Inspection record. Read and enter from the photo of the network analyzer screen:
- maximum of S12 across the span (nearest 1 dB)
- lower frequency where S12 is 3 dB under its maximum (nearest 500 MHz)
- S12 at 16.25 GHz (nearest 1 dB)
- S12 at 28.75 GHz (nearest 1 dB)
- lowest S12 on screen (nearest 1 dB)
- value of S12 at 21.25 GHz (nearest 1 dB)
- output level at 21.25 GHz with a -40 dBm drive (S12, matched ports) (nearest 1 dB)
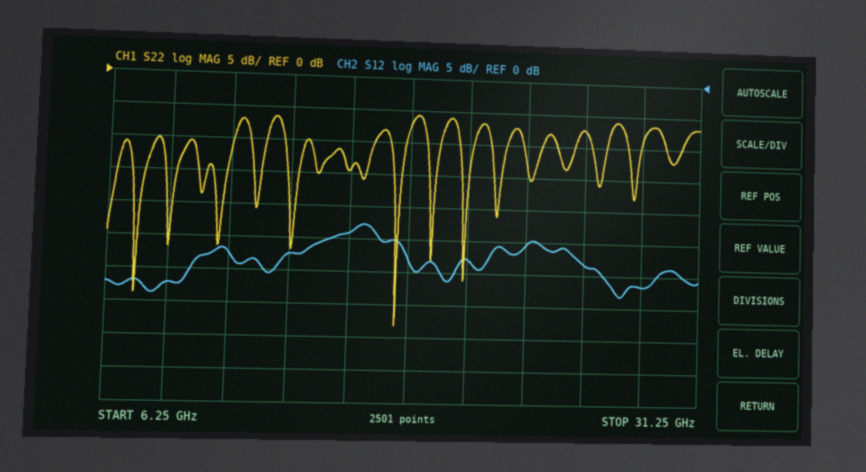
-23 dB
15.0 GHz
-24 dB
-32 dB
-34 dB
-28 dB
-68 dBm
